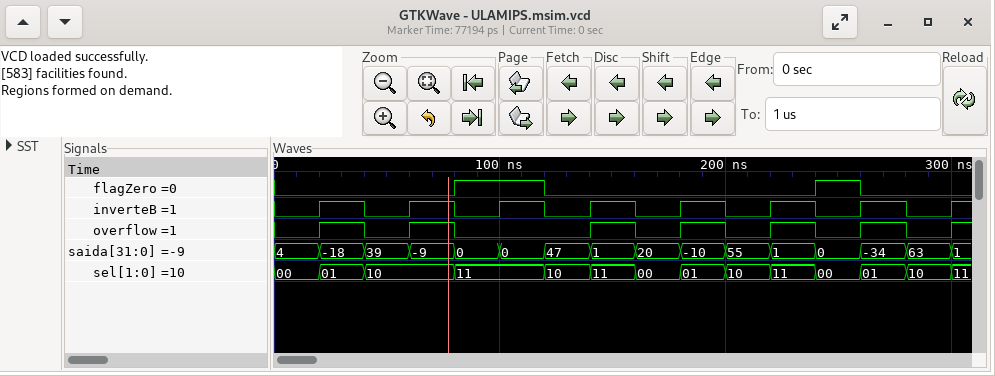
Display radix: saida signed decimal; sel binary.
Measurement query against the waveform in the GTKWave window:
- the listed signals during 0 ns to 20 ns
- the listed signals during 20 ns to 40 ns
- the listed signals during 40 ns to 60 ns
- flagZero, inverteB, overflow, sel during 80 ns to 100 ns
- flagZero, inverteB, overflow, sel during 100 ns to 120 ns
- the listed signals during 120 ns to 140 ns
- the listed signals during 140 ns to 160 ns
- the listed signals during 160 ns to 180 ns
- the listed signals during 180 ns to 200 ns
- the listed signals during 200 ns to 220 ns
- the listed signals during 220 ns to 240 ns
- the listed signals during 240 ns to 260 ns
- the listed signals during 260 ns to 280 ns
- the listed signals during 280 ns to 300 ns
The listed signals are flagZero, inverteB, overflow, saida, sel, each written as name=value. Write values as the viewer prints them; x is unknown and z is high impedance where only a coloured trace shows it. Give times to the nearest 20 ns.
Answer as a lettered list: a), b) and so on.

a) flagZero=0, inverteB=0, overflow=0, saida=4, sel=00
b) flagZero=0, inverteB=1, overflow=1, saida=-18, sel=01
c) flagZero=0, inverteB=0, overflow=0, saida=39, sel=10
d) flagZero=1, inverteB=0, overflow=0, sel=11
e) flagZero=1, inverteB=1, overflow=0, sel=11
f) flagZero=0, inverteB=0, overflow=0, saida=47, sel=10
g) flagZero=0, inverteB=1, overflow=1, saida=1, sel=11
h) flagZero=0, inverteB=0, overflow=0, saida=20, sel=00
i) flagZero=0, inverteB=1, overflow=1, saida=-10, sel=01
j) flagZero=0, inverteB=0, overflow=0, saida=55, sel=10
k) flagZero=0, inverteB=1, overflow=1, saida=1, sel=11
l) flagZero=1, inverteB=0, overflow=0, saida=0, sel=00
m) flagZero=0, inverteB=1, overflow=1, saida=-34, sel=01
n) flagZero=0, inverteB=0, overflow=0, saida=63, sel=10
